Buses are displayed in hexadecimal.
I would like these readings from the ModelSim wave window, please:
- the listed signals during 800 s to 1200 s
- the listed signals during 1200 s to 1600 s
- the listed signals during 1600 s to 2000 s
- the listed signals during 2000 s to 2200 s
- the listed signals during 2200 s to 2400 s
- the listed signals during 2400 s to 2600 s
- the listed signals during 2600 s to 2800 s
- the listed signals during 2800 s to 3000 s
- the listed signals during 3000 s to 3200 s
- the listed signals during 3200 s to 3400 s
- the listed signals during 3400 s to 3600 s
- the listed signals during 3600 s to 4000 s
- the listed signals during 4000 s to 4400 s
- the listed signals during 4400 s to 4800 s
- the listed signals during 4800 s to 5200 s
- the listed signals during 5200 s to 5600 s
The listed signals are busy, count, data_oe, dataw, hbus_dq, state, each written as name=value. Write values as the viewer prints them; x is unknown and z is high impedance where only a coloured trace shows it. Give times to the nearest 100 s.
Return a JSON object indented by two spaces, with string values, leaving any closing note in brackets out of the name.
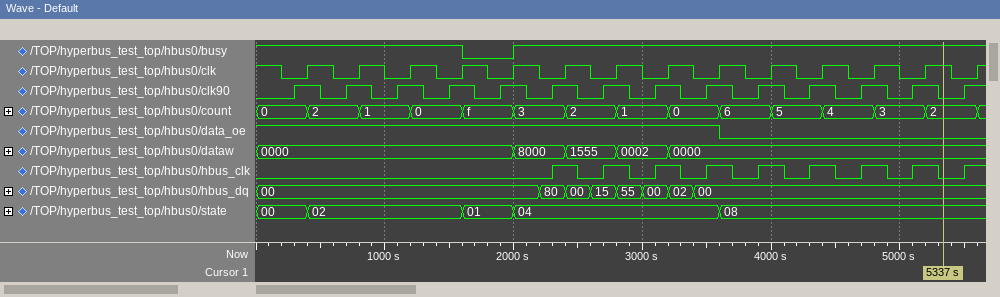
{
  "the listed signals during 800 s to 1200 s": "busy=1, count=1, data_oe=1, dataw=0000, hbus_dq=00, state=02",
  "the listed signals during 1200 s to 1600 s": "busy=1, count=0, data_oe=1, dataw=0000, hbus_dq=00, state=02",
  "the listed signals during 1600 s to 2000 s": "busy=0, count=f, data_oe=1, dataw=0000, hbus_dq=00, state=01",
  "the listed signals during 2000 s to 2200 s": "busy=1, count=3, data_oe=1, dataw=8000, hbus_dq=00, state=04",
  "the listed signals during 2200 s to 2400 s": "busy=1, count=3, data_oe=1, dataw=8000, hbus_dq=80, state=04",
  "the listed signals during 2400 s to 2600 s": "busy=1, count=2, data_oe=1, dataw=1555, hbus_dq=00, state=04",
  "the listed signals during 2600 s to 2800 s": "busy=1, count=2, data_oe=1, dataw=1555, hbus_dq=15, state=04",
  "the listed signals during 2800 s to 3000 s": "busy=1, count=1, data_oe=1, dataw=0002, hbus_dq=55, state=04",
  "the listed signals during 3000 s to 3200 s": "busy=1, count=1, data_oe=1, dataw=0002, hbus_dq=00, state=04",
  "the listed signals during 3200 s to 3400 s": "busy=1, count=0, data_oe=1, dataw=0000, hbus_dq=02, state=04",
  "the listed signals during 3400 s to 3600 s": "busy=1, count=0, data_oe=1, dataw=0000, hbus_dq=00, state=04",
  "the listed signals during 3600 s to 4000 s": "busy=1, count=6, data_oe=0, dataw=0000, hbus_dq=00, state=08",
  "the listed signals during 4000 s to 4400 s": "busy=1, count=5, data_oe=0, dataw=0000, hbus_dq=00, state=08",
  "the listed signals during 4400 s to 4800 s": "busy=1, count=4, data_oe=0, dataw=0000, hbus_dq=00, state=08",
  "the listed signals during 4800 s to 5200 s": "busy=1, count=3, data_oe=0, dataw=0000, hbus_dq=00, state=08",
  "the listed signals during 5200 s to 5600 s": "busy=1, count=2, data_oe=0, dataw=0000, hbus_dq=00, state=08"
}
